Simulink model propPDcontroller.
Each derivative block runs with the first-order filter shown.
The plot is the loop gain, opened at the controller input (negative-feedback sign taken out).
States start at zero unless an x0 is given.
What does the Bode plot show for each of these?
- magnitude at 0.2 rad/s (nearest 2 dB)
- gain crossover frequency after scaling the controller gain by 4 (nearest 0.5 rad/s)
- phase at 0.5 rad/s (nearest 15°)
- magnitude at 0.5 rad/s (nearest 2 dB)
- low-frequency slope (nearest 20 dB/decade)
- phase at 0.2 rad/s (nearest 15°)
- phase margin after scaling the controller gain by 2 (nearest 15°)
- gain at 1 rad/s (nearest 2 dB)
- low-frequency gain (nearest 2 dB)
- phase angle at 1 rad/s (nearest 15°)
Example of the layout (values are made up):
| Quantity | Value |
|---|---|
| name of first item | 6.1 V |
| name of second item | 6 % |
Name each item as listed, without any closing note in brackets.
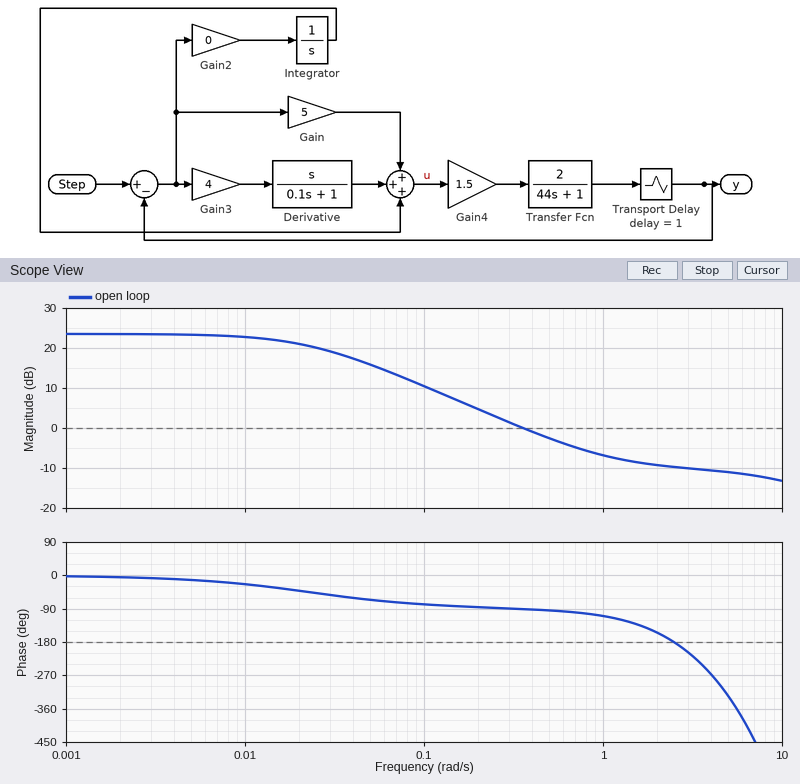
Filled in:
| Quantity | Value |
|---|---|
| magnitude at 0.2 rad/s | 4 dB |
| gain crossover frequency after scaling the controller gain by 4 | 7.5 rad/s |
| phase at 0.5 rad/s | -90° |
| magnitude at 0.5 rad/s | -2 dB |
| low-frequency slope | 0 dB/decade |
| phase at 0.2 rad/s | -90° |
| phase margin after scaling the controller gain by 2 | 75° |
| gain at 1 rad/s | -6 dB |
| low-frequency gain | 24 dB |
| phase angle at 1 rad/s | -105° |
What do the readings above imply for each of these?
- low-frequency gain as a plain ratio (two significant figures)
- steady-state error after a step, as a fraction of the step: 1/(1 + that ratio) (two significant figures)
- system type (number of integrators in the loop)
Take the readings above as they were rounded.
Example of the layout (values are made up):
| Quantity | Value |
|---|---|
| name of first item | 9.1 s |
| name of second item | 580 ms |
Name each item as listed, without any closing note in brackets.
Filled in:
| Quantity | Value |
|---|---|
| low-frequency gain as a plain ratio | 16 |
| steady-state error after a step, as a fraction of the step: 1/(1 + that ratio) | 0.059 |
| system type | 0 |
